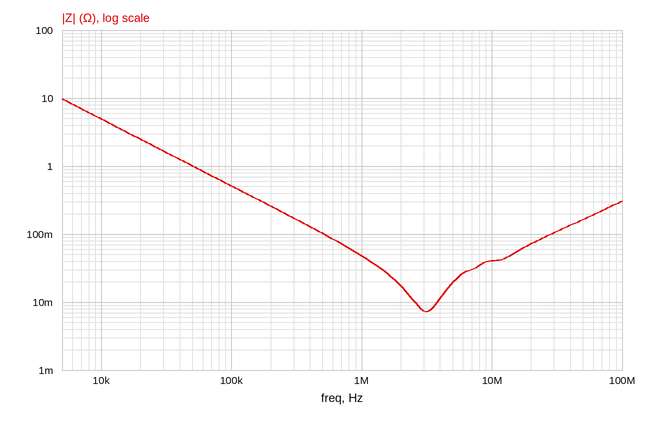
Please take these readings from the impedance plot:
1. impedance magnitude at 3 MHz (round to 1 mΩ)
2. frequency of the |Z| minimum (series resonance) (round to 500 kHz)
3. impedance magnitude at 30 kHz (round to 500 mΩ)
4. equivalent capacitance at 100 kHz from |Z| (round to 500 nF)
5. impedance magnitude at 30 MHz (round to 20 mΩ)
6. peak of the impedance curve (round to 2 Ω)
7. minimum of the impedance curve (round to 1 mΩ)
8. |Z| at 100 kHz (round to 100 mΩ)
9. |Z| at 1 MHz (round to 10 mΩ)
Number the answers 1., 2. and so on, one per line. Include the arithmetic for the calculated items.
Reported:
1. 7 mΩ
2. 3.0 MHz
3. 1.5 Ω
4. C = 1/(2π × 100 kHz × 500 mΩ) ≈ 3.18 µF, so 3.0 µF to the nearest 500 nF
5. 100 mΩ
6. 10 Ω
7. 7 mΩ
8. 500 mΩ
9. 50 mΩ
